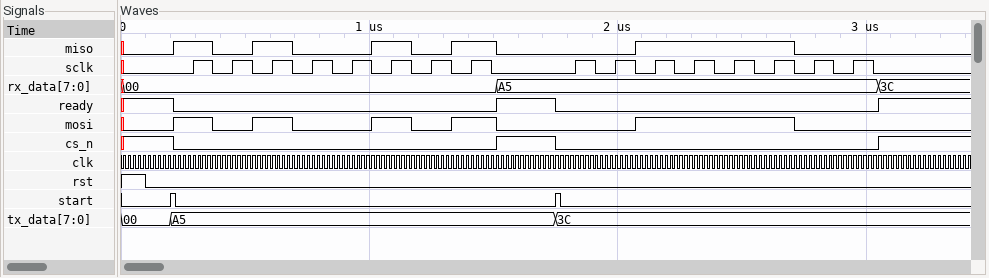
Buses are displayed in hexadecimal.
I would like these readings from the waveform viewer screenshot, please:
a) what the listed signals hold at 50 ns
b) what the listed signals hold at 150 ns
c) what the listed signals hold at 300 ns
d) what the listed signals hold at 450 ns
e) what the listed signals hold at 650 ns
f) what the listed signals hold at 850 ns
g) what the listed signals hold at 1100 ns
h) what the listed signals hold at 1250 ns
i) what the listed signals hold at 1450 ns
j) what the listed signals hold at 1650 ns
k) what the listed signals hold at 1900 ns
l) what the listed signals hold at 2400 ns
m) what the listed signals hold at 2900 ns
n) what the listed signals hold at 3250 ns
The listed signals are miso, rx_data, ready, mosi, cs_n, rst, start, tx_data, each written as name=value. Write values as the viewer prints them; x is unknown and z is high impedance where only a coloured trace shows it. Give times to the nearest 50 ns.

miso=0, rx_data=00, ready=1, mosi=0, cs_n=1, rst=1, start=0, tx_data=00
miso=0, rx_data=00, ready=1, mosi=0, cs_n=1, rst=0, start=0, tx_data=00
miso=1, rx_data=00, ready=0, mosi=1, cs_n=0, rst=0, start=0, tx_data=A5
miso=0, rx_data=00, ready=0, mosi=0, cs_n=0, rst=0, start=0, tx_data=A5
miso=1, rx_data=00, ready=0, mosi=1, cs_n=0, rst=0, start=0, tx_data=A5
miso=0, rx_data=00, ready=0, mosi=0, cs_n=0, rst=0, start=0, tx_data=A5
miso=1, rx_data=00, ready=0, mosi=1, cs_n=0, rst=0, start=0, tx_data=A5
miso=0, rx_data=00, ready=0, mosi=0, cs_n=0, rst=0, start=0, tx_data=A5
miso=1, rx_data=00, ready=0, mosi=1, cs_n=0, rst=0, start=0, tx_data=A5
miso=0, rx_data=A5, ready=1, mosi=0, cs_n=1, rst=0, start=0, tx_data=A5
miso=0, rx_data=A5, ready=0, mosi=0, cs_n=0, rst=0, start=0, tx_data=3C
miso=1, rx_data=A5, ready=0, mosi=1, cs_n=0, rst=0, start=0, tx_data=3C
miso=0, rx_data=A5, ready=0, mosi=0, cs_n=0, rst=0, start=0, tx_data=3C
miso=0, rx_data=3C, ready=1, mosi=0, cs_n=1, rst=0, start=0, tx_data=3C
